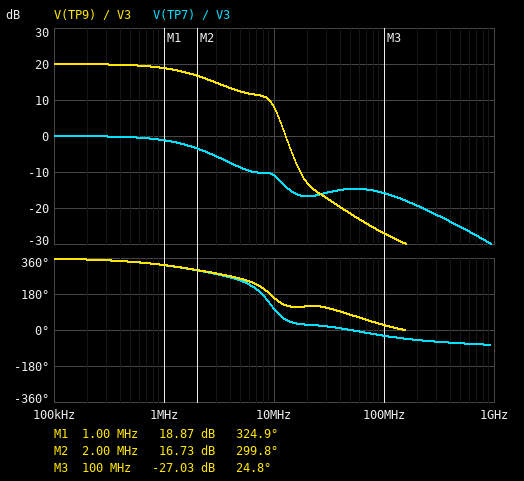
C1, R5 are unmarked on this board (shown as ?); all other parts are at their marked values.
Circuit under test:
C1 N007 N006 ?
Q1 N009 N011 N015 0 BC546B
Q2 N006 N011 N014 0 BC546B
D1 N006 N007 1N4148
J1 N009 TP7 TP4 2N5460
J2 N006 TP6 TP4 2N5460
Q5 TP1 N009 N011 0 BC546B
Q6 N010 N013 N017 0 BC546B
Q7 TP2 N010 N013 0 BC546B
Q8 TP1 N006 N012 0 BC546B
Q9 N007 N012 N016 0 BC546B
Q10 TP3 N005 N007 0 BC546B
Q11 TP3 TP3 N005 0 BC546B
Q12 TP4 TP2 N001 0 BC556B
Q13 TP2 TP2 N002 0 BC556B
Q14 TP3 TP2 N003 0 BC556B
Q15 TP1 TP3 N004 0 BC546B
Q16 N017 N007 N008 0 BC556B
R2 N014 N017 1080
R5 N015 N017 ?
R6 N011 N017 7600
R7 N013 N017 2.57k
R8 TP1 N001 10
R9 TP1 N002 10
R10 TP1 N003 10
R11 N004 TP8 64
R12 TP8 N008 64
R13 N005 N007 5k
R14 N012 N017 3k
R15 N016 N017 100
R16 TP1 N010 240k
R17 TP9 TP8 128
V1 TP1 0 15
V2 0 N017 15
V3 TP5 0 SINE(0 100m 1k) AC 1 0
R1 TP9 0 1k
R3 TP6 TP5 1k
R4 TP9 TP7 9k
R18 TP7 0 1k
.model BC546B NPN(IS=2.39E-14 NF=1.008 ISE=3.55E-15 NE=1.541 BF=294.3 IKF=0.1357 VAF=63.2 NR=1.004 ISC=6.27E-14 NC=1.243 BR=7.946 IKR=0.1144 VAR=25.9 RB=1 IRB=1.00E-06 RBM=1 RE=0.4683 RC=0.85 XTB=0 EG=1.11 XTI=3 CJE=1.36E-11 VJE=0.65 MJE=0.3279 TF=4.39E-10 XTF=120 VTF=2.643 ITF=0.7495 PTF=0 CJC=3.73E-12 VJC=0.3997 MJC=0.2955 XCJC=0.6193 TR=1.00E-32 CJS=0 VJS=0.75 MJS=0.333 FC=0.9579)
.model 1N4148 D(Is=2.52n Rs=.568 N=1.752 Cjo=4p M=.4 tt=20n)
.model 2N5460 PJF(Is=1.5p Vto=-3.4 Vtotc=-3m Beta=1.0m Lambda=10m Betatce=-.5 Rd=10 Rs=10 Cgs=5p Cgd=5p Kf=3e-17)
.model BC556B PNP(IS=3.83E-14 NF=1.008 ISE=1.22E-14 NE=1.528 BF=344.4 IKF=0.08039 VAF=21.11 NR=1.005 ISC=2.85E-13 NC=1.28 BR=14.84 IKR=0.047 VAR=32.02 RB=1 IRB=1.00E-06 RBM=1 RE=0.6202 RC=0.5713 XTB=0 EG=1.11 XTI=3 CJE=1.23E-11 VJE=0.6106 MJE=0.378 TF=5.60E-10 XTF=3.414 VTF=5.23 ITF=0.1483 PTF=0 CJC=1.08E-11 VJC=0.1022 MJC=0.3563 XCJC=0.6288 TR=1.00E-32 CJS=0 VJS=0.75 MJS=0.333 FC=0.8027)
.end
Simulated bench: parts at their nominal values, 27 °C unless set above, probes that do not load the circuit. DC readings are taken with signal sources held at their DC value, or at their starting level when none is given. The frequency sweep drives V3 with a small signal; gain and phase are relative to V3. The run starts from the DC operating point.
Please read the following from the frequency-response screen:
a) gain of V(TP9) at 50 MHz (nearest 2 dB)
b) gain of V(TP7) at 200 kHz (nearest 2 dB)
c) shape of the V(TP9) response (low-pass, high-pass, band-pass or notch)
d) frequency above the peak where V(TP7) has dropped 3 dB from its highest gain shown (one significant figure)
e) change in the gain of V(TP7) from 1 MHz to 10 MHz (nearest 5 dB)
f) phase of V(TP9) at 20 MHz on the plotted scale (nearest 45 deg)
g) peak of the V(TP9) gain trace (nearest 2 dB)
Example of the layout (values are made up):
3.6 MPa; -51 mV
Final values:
-22 dB; 0 dB; low-pass; 2 MHz; -10 dB; 135 deg; 20 dB
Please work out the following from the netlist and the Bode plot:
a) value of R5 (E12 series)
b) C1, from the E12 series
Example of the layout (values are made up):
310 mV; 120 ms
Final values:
1.8 kΩ; 8.2 pF
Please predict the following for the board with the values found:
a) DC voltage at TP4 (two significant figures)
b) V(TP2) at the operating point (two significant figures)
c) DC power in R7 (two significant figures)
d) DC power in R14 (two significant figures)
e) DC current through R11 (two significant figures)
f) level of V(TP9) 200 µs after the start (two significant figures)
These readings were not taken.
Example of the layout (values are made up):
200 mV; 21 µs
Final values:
-2.9 V; 14 V; 130 µW; 140 µW; 1.1 mA; 1.9 V
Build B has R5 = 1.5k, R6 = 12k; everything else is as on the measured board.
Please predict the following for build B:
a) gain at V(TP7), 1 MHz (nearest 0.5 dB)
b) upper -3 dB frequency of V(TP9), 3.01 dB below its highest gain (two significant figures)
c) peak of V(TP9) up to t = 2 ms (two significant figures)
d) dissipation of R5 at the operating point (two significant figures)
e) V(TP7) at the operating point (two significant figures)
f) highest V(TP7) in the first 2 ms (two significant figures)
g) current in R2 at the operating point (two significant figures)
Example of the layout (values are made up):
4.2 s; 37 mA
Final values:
-1.5 dB; 1.7 MHz; 1.6 V; 41 µW; 62 mV; 160 mV; 220 µA
